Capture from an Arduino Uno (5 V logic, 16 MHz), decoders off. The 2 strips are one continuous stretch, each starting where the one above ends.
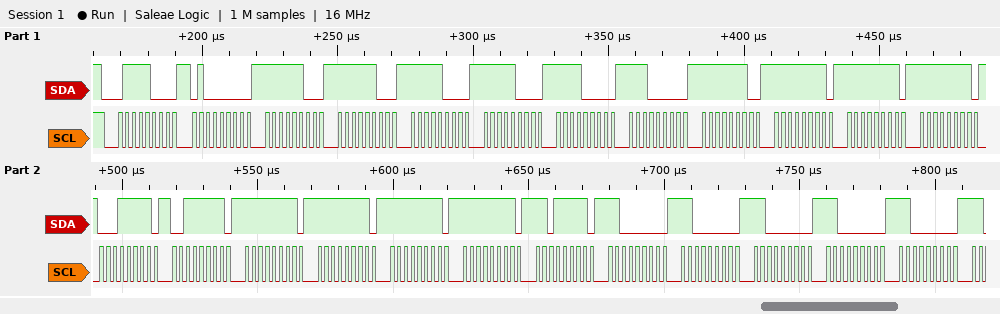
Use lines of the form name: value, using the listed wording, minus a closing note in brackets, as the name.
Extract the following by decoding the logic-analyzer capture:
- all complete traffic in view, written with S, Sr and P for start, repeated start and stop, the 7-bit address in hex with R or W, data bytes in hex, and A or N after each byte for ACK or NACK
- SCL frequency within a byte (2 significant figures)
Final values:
all complete traffic in view, written with S, Sr and P for start, repeated start and stop, the 7-bit address in hex with R or W, data bytes in hex, and A or N after each byte for ACK or NACK: S 3CW A 40 A FC A FC A F8 A F8 A F0 A E0 A FE A FF A FF A FF A 1F A 3F A FF A FF A FF A FF A DF A C0 A C0 A C0 A C0 A C0 A
SCL frequency within a byte: 400 kHz
